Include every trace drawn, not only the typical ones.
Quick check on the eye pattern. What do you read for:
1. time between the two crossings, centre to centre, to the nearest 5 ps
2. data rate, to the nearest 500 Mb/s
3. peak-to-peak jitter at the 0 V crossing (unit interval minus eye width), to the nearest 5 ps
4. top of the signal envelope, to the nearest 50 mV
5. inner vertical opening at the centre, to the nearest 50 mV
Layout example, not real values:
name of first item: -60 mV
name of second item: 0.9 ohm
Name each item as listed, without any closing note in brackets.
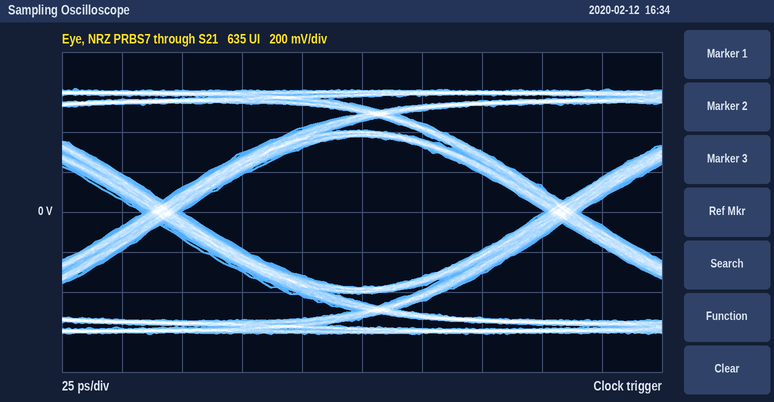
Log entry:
time between the two crossings, centre to centre, to the nearest 5 ps: 165 ps
data rate, to the nearest 500 Mb/s: 6.0 Gb/s
peak-to-peak jitter at the 0 V crossing (unit interval minus eye width), to the nearest 5 ps: 15 ps
top of the signal envelope, to the nearest 50 mV: 600 mV
inner vertical opening at the centre, to the nearest 50 mV: 750 mV
